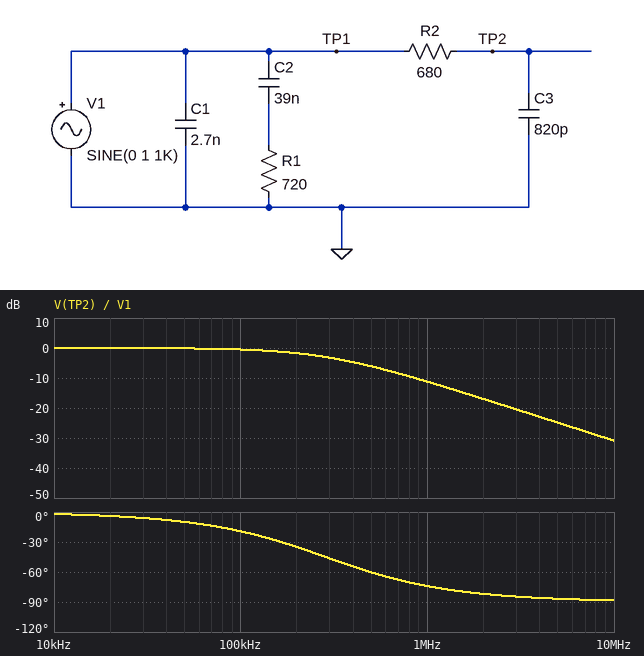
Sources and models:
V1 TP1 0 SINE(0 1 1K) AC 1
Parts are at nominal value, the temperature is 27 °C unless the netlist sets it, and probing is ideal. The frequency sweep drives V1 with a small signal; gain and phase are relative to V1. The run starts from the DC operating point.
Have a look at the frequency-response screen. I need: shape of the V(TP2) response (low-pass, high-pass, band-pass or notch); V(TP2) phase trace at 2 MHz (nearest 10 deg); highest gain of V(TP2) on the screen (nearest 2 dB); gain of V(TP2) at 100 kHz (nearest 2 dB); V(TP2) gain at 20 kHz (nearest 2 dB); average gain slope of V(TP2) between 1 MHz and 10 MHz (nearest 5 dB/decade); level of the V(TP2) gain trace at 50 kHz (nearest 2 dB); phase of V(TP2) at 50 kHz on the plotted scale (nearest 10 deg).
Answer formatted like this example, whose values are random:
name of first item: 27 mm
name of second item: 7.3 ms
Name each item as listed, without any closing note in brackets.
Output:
shape of the V(TP2) response: low-pass
V(TP2) phase trace at 2 MHz: -80 deg
highest gain of V(TP2) on the screen: 0 dB
gain of V(TP2) at 100 kHz: 0 dB
V(TP2) gain at 20 kHz: 0 dB
average gain slope of V(TP2) between 1 MHz and 10 MHz: -20 dB/decade
level of the V(TP2) gain trace at 50 kHz: 0 dB
phase of V(TP2) at 50 kHz on the plotted scale: -10 deg
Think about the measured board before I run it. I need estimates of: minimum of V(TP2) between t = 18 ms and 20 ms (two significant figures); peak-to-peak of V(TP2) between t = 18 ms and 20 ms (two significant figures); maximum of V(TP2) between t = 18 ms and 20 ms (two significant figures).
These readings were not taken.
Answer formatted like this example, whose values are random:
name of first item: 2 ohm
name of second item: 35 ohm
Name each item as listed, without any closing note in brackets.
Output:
minimum of V(TP2) between t = 18 ms and 20 ms: -1.0 V
peak-to-peak of V(TP2) between t = 18 ms and 20 ms: 2.0 V
maximum of V(TP2) between t = 18 ms and 20 ms: 1.0 V
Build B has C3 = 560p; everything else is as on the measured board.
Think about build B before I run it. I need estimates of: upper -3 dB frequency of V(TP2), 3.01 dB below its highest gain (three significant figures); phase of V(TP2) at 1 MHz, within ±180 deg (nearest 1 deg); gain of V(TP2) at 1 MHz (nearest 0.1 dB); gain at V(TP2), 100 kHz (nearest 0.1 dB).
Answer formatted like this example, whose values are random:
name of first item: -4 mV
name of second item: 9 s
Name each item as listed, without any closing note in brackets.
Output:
upper -3 dB frequency of V(TP2), 3.01 dB below its highest gain: 418 kHz
phase of V(TP2) at 1 MHz, within ±180 deg: -67 deg
gain of V(TP2) at 1 MHz: -8.3 dB
gain at V(TP2), 100 kHz: -0.2 dB
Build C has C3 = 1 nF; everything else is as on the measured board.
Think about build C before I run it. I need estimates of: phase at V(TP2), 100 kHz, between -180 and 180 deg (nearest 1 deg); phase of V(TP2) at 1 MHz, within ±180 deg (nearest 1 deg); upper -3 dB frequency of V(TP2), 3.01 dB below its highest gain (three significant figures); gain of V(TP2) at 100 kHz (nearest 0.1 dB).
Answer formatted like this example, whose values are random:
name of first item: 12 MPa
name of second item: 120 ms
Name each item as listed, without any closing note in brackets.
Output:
phase at V(TP2), 100 kHz, between -180 and 180 deg: -23 deg
phase of V(TP2) at 1 MHz, within ±180 deg: -77 deg
upper -3 dB frequency of V(TP2), 3.01 dB below its highest gain: 234 kHz
gain of V(TP2) at 100 kHz: -0.7 dB
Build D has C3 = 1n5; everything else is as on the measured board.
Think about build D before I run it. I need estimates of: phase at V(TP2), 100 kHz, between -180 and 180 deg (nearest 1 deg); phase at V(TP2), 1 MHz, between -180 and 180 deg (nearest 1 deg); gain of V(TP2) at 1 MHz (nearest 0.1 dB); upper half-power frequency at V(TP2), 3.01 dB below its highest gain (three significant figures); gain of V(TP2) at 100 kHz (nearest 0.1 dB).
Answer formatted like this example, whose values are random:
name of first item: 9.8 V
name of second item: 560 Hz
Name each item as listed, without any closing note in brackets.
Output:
phase at V(TP2), 100 kHz, between -180 and 180 deg: -33 deg
phase at V(TP2), 1 MHz, between -180 and 180 deg: -81 deg
gain of V(TP2) at 1 MHz: -16.2 dB
upper half-power frequency at V(TP2), 3.01 dB below its highest gain: 156 kHz
gain of V(TP2) at 100 kHz: -1.5 dB
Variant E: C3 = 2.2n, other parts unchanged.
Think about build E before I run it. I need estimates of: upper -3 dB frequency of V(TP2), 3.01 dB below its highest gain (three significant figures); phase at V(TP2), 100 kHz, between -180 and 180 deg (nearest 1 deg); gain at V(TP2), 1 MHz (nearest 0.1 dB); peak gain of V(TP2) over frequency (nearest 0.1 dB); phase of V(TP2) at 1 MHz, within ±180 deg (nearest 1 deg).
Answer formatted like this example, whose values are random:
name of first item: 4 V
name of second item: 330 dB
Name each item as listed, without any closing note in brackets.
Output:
upper -3 dB frequency of V(TP2), 3.01 dB below its highest gain: 106 kHz
phase at V(TP2), 100 kHz, between -180 and 180 deg: -43 deg
gain at V(TP2), 1 MHz: -19.5 dB
peak gain of V(TP2) over frequency: 0 dB
phase of V(TP2) at 1 MHz, within ±180 deg: -84 deg
